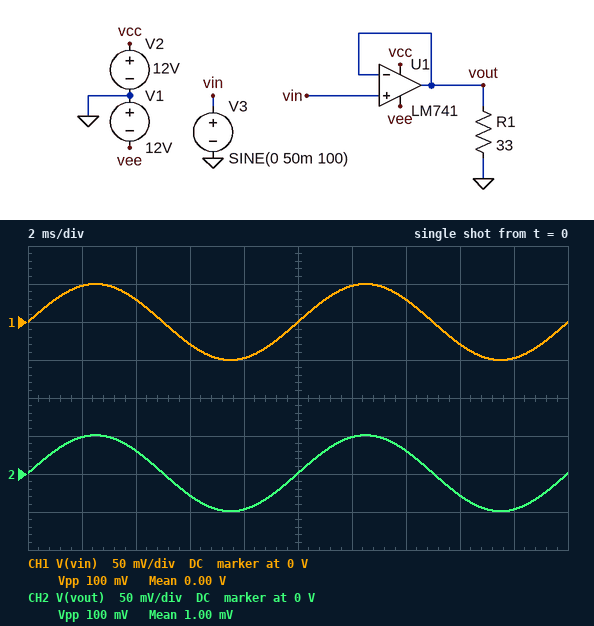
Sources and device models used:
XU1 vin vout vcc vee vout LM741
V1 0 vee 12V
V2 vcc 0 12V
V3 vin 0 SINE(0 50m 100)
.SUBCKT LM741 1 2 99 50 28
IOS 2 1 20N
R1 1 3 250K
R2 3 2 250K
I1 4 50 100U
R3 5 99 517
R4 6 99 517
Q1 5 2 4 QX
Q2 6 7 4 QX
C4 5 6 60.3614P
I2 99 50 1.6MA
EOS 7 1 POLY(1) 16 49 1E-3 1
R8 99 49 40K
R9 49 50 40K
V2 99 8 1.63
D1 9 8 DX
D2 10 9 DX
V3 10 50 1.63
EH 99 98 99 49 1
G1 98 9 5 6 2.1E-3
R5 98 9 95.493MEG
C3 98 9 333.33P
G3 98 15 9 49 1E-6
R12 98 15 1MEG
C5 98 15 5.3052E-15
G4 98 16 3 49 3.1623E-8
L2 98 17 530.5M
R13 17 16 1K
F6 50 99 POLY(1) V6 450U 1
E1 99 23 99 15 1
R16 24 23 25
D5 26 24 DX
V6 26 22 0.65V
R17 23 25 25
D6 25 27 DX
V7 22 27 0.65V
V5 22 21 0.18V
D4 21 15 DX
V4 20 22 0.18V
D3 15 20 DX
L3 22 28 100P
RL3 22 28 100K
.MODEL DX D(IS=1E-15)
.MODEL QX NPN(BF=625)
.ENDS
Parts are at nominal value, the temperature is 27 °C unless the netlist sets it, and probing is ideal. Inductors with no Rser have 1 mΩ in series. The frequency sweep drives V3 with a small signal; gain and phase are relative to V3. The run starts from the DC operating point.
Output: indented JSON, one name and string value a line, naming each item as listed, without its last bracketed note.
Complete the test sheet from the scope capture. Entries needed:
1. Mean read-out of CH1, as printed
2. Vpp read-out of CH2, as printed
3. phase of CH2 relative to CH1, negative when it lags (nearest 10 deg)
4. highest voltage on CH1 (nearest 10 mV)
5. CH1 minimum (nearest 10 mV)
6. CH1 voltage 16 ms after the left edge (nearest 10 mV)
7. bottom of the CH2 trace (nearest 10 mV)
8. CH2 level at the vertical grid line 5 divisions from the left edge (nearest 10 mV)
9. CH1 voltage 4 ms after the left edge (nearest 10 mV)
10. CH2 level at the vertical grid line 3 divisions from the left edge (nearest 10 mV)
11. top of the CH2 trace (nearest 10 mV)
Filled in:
{
  "Mean read-out of CH1, as printed": "0.00 V",
  "Vpp read-out of CH2, as printed": "100 mV",
  "phase of CH2 relative to CH1, negative when it lags": "0 deg",
  "highest voltage on CH1": "50 mV",
  "CH1 minimum": "-50 mV",
  "CH1 voltage 16 ms after the left edge": "-30 mV",
  "bottom of the CH2 trace": "-50 mV",
  "CH2 level at the vertical grid line 5 divisions from the left edge": "0 V",
  "CH1 voltage 4 ms after the left edge": "30 mV",
  "CH2 level at the vertical grid line 3 divisions from the left edge": "-30 mV",
  "top of the CH2 trace": "50 mV"
}
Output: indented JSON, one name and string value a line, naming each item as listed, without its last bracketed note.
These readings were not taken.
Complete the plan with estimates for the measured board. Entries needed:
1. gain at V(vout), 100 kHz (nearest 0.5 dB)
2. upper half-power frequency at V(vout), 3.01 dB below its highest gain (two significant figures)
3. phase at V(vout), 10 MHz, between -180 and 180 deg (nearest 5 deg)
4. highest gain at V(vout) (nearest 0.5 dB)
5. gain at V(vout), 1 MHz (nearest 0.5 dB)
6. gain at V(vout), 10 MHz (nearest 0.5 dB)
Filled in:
{
  "gain at V(vout), 100 kHz": "-1.5 dB",
  "upper half-power frequency at V(vout), 3.01 dB below its highest gain": "170 kHz",
  "phase at V(vout), 10 MHz, between -180 and 180 deg": "-155 deg",
  "highest gain at V(vout)": "0 dB",
  "gain at V(vout), 1 MHz": "-16.5 dB",
  "gain at V(vout), 10 MHz": "-48.0 dB"
}
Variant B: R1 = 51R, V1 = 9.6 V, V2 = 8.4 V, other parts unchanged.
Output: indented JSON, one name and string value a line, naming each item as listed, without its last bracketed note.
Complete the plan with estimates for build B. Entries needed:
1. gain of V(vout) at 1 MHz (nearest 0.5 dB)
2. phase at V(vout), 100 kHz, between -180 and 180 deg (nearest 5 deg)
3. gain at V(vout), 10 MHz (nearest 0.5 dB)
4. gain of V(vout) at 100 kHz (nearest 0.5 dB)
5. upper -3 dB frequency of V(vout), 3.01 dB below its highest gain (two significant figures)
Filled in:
{
  "gain of V(vout) at 1 MHz": "-13.0 dB",
  "phase at V(vout), 100 kHz, between -180 and 180 deg": "-25 deg",
  "gain at V(vout), 10 MHz": "-45.0 dB",
  "gain of V(vout) at 100 kHz": "-0.5 dB",
  "upper -3 dB frequency of V(vout), 3.01 dB below its highest gain": "250 kHz"
}
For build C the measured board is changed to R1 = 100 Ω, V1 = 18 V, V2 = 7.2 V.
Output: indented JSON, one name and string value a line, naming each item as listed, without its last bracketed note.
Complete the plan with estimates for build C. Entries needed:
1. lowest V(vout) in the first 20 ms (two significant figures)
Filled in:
{
  "lowest V(vout) in the first 20 ms": "-49 mV"
}
